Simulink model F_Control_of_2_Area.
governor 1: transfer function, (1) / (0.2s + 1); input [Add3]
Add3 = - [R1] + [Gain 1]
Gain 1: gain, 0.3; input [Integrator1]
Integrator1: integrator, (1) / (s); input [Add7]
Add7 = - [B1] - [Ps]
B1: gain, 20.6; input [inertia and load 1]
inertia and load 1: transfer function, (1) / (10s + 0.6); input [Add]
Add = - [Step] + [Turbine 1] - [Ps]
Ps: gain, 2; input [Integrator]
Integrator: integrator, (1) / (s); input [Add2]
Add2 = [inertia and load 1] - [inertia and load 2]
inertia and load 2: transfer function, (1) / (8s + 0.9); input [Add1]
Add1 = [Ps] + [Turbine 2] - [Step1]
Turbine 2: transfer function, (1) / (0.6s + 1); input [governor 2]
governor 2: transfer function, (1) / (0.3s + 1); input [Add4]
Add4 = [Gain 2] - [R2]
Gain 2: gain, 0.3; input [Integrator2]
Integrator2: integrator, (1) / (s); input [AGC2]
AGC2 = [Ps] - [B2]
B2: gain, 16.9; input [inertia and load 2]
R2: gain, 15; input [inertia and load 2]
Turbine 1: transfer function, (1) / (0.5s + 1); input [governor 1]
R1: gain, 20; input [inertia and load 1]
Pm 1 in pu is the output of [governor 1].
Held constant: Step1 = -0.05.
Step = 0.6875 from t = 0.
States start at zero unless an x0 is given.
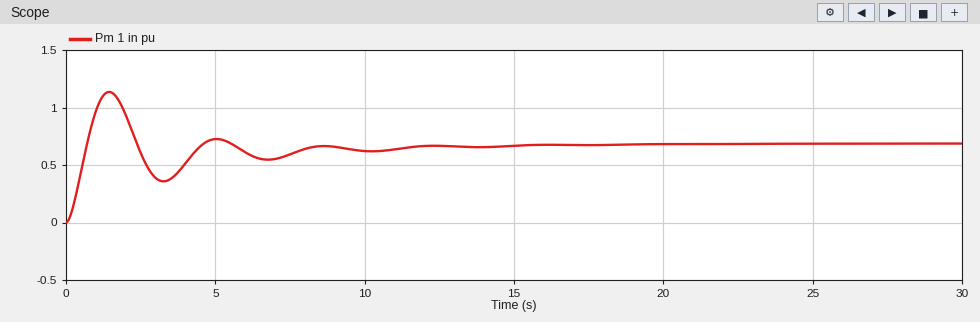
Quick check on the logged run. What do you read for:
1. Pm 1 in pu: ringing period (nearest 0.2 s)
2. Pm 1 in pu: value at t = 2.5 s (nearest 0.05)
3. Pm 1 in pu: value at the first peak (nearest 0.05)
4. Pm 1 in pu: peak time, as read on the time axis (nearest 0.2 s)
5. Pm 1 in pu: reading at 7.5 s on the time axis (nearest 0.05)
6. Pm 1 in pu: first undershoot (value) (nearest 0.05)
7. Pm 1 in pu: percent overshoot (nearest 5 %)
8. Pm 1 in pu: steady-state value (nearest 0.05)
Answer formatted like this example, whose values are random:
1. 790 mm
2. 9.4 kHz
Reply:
1. 3.6 s
2. 0.60
3. 1.15
4. 1.4 s
5. 0.60
6. 0.35
7. 65 %
8. 0.70
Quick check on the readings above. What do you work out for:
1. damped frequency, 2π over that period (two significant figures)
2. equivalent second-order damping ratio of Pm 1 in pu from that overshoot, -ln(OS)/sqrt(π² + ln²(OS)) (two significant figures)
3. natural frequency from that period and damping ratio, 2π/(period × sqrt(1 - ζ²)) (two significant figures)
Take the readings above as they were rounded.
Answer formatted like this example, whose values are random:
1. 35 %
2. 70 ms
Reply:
1. 1.7 rad/s
2. 0.14
3. 1.8 rad/s
